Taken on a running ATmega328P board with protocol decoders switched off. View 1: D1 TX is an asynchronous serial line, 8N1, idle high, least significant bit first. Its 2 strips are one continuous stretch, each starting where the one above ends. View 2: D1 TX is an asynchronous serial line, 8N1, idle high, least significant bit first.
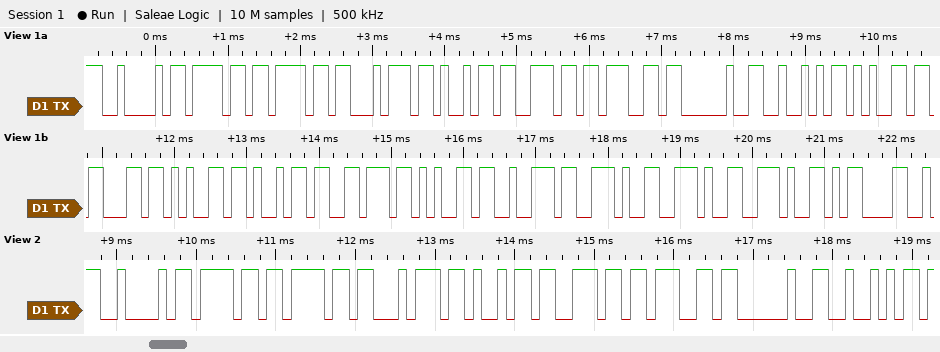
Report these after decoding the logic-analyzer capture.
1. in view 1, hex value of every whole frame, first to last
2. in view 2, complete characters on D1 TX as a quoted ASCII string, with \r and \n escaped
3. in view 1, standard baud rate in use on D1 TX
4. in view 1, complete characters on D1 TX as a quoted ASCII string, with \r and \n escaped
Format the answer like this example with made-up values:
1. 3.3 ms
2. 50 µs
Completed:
1. 42 6F 6F 74 69 6E 67 20 52 65 63 65 69 76 65 72 2E 2E 2E 0D
2. "Booting R"
3. 9600 baud
4. "Booting Receiver...\r"
